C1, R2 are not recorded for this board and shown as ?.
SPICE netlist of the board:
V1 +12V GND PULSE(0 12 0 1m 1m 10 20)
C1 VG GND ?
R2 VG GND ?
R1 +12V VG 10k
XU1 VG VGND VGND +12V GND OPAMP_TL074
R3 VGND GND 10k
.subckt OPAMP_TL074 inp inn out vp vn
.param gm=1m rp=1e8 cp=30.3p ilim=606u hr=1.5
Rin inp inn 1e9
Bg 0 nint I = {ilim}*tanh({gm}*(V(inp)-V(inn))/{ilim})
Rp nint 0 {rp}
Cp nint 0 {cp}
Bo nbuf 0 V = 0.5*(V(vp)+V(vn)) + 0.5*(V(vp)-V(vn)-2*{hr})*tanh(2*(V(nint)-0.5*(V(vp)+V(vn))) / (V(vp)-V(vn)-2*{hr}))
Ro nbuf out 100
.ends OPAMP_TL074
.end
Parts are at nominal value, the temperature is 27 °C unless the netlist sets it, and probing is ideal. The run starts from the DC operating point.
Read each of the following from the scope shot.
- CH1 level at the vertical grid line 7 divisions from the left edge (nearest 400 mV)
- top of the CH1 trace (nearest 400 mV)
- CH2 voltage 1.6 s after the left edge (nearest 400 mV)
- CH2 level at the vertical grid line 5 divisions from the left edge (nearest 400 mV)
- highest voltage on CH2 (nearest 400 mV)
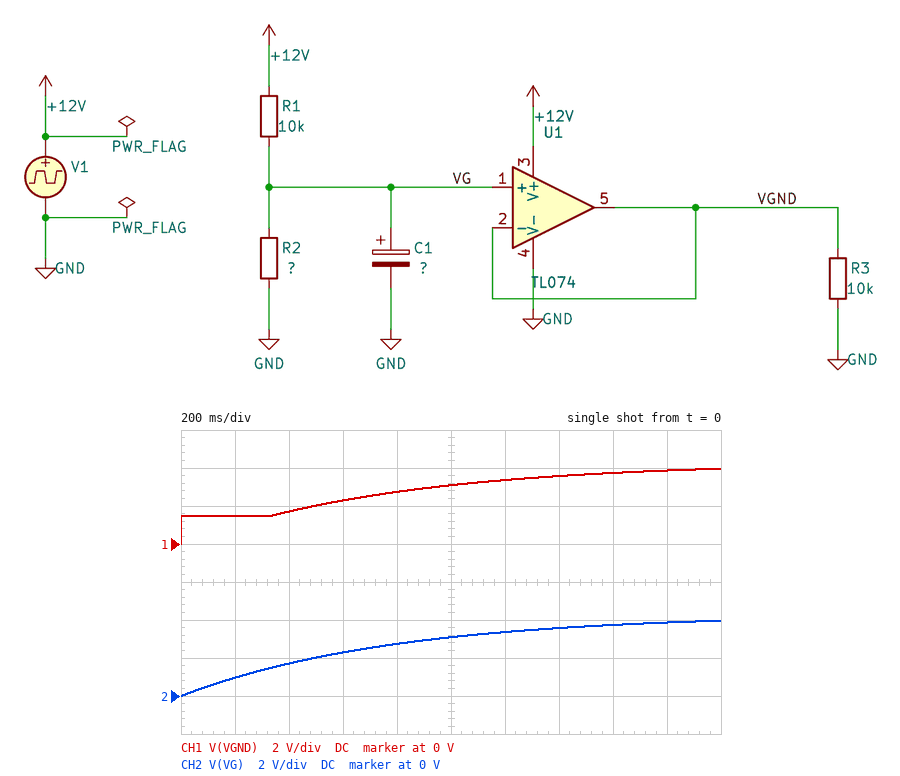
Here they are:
3.6 V
4.0 V
3.6 V
3.2 V
4.0 V
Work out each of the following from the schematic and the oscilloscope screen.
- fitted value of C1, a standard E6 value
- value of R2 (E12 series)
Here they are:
220 µF
5.6 kΩ
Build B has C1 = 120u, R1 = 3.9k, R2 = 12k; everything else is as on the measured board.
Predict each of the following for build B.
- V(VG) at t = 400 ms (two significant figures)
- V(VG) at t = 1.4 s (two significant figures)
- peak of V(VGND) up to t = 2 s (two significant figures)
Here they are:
6.1 V
8.9 V
9.0 V
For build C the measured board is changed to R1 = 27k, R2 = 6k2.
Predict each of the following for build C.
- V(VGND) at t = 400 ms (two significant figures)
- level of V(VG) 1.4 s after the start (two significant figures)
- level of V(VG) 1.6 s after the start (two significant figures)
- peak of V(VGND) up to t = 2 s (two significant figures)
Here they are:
1.5 V
1.6 V
1.7 V
1.9 V
